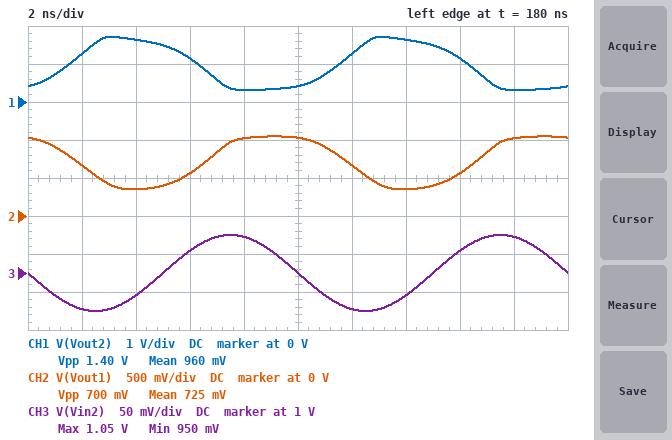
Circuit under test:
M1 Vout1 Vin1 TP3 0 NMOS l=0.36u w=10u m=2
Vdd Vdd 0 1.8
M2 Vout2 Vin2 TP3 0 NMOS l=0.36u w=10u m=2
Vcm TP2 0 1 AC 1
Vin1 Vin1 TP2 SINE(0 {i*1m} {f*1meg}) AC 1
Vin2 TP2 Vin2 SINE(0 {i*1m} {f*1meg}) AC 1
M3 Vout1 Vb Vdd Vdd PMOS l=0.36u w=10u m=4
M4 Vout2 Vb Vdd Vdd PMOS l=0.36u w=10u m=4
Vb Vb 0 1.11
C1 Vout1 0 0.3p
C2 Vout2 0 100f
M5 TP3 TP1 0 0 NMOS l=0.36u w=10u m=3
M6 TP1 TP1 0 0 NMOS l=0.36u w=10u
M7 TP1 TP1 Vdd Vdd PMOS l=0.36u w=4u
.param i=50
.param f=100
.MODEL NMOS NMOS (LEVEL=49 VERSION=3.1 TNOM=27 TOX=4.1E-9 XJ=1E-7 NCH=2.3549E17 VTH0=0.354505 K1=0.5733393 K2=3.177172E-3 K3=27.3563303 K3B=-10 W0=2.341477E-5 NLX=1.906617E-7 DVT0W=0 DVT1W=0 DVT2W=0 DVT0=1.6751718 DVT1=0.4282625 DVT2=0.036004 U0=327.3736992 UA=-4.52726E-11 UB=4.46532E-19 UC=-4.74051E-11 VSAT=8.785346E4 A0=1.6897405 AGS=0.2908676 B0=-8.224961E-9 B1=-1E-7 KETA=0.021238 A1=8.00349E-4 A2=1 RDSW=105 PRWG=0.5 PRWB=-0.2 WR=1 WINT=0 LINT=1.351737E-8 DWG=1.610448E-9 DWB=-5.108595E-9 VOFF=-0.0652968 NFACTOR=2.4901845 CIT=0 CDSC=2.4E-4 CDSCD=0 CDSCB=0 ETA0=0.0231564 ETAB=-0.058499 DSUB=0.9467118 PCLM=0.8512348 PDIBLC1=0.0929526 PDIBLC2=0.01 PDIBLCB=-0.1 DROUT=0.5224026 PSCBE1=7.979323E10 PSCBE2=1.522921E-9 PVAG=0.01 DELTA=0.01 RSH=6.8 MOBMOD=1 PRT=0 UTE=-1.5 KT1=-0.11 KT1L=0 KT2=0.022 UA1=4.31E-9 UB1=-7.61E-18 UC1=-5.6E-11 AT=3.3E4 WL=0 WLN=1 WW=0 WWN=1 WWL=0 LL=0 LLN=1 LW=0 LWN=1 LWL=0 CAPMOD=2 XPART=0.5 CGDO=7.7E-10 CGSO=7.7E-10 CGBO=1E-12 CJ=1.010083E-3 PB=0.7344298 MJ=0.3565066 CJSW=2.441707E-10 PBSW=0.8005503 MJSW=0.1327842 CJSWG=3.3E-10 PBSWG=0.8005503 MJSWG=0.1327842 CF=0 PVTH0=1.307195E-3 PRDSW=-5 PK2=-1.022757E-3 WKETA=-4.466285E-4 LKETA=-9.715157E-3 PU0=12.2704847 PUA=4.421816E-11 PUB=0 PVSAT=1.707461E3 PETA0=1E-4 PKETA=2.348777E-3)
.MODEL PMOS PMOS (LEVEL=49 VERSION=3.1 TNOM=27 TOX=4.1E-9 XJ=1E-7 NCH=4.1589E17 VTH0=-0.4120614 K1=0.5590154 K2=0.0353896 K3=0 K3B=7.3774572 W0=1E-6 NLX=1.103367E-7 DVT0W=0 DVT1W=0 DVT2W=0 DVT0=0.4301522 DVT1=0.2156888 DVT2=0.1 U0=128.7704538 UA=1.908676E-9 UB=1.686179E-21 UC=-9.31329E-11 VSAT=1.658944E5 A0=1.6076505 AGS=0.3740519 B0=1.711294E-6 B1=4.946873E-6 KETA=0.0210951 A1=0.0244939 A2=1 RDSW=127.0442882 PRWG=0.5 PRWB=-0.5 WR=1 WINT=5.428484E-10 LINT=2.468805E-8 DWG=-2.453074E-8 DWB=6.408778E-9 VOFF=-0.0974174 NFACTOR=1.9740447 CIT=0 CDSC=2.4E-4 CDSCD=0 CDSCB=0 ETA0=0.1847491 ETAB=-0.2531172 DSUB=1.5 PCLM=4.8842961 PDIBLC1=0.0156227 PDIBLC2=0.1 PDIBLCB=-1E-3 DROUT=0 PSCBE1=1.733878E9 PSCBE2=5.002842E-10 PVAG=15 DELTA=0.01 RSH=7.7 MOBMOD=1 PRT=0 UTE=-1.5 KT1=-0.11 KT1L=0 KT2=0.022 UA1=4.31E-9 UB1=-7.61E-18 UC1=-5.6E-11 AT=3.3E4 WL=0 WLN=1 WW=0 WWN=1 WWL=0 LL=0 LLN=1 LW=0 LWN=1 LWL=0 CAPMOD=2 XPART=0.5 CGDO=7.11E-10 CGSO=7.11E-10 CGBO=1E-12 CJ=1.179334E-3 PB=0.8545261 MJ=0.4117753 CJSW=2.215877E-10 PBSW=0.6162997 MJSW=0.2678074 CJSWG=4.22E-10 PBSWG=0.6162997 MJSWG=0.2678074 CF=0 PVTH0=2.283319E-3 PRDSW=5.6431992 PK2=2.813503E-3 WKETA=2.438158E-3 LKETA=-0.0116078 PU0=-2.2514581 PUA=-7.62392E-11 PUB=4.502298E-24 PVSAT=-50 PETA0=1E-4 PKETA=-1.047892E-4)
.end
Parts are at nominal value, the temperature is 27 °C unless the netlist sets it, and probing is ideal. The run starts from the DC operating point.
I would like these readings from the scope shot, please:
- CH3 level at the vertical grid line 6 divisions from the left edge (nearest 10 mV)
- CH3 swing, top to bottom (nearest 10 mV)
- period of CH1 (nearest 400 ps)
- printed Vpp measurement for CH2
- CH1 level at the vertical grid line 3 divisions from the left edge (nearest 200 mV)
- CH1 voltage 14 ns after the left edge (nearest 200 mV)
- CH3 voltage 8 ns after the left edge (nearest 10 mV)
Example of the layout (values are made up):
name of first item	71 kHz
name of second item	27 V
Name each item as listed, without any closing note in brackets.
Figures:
CH3 level at the vertical grid line 6 divisions from the left edge	950 mV
CH3 swing, top to bottom	100 mV
period of CH1	10.0 ns
printed Vpp measurement for CH2	700 mV
CH1 level at the vertical grid line 3 divisions from the left edge	1.2 V
CH1 voltage 14 ns after the left edge	1.6 V
CH3 voltage 8 ns after the left edge	1.05 V
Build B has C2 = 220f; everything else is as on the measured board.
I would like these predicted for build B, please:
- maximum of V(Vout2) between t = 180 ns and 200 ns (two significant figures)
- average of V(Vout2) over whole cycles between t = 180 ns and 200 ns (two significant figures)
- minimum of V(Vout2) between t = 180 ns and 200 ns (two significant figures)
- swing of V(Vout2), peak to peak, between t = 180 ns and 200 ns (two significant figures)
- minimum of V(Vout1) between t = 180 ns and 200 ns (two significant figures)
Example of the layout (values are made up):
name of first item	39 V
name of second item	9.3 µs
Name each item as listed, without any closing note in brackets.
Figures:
maximum of V(Vout2) between t = 180 ns and 200 ns	1.6 V
average of V(Vout2) over whole cycles between t = 180 ns and 200 ns	990 mV
minimum of V(Vout2) between t = 180 ns and 200 ns	390 mV
swing of V(Vout2), peak to peak, between t = 180 ns and 200 ns	1.2 V
minimum of V(Vout1) between t = 180 ns and 200 ns	440 mV
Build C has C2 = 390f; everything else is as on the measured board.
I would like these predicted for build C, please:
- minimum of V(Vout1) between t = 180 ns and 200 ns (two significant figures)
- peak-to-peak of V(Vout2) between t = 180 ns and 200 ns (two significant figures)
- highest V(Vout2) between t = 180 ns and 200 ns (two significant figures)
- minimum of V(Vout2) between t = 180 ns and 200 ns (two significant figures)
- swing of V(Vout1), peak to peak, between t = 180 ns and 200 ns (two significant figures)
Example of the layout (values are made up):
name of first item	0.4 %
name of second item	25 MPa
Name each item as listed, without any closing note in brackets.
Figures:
minimum of V(Vout1) between t = 180 ns and 200 ns	480 mV
peak-to-peak of V(Vout2) between t = 180 ns and 200 ns	780 mV
highest V(Vout2) between t = 180 ns and 200 ns	1.4 V
minimum of V(Vout2) between t = 180 ns and 200 ns	580 mV
swing of V(Vout1), peak to peak, between t = 180 ns and 200 ns	1.0 V
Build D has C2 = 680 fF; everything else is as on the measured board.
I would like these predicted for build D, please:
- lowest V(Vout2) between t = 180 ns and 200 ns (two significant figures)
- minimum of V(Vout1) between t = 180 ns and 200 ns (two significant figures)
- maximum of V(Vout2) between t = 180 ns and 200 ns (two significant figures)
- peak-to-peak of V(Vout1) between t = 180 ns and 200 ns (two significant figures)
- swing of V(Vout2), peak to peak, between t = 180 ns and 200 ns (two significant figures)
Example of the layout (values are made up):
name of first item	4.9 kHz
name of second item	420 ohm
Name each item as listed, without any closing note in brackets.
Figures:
lowest V(Vout2) between t = 180 ns and 200 ns	730 mV
minimum of V(Vout1) between t = 180 ns and 200 ns	490 mV
maximum of V(Vout2) between t = 180 ns and 200 ns	1.2 V
peak-to-peak of V(Vout1) between t = 180 ns and 200 ns	1.0 V
swing of V(Vout2), peak to peak, between t = 180 ns and 200 ns	480 mV
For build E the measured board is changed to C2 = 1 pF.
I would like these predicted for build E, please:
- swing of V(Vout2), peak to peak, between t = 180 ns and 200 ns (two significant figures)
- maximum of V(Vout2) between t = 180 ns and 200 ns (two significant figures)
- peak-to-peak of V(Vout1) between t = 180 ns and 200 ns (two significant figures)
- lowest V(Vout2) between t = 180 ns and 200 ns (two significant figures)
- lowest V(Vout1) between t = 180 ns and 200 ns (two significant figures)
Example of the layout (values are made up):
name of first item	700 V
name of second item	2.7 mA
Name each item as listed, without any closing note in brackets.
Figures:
swing of V(Vout2), peak to peak, between t = 180 ns and 200 ns	330 mV
maximum of V(Vout2) between t = 180 ns and 200 ns	1.1 V
peak-to-peak of V(Vout1) between t = 180 ns and 200 ns	1.0 V
lowest V(Vout2) between t = 180 ns and 200 ns	800 mV
lowest V(Vout1) between t = 180 ns and 200 ns	490 mV
